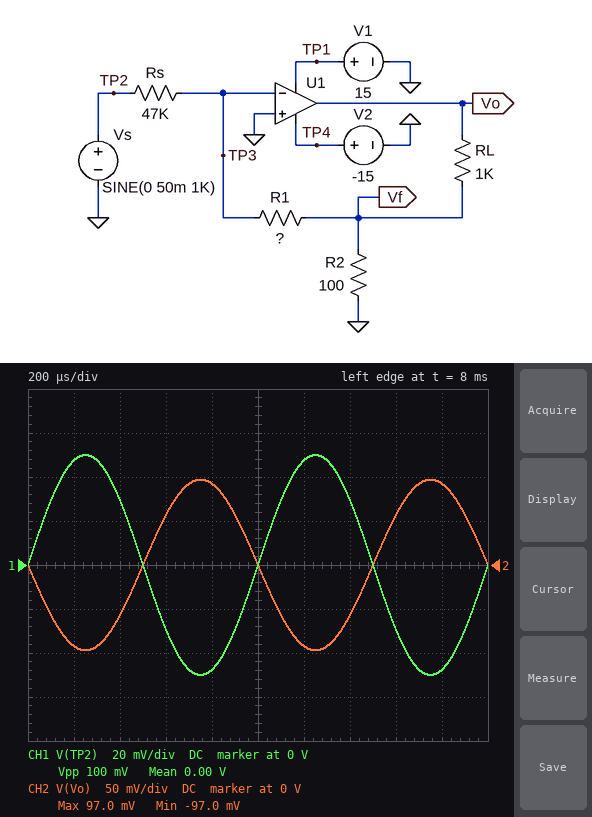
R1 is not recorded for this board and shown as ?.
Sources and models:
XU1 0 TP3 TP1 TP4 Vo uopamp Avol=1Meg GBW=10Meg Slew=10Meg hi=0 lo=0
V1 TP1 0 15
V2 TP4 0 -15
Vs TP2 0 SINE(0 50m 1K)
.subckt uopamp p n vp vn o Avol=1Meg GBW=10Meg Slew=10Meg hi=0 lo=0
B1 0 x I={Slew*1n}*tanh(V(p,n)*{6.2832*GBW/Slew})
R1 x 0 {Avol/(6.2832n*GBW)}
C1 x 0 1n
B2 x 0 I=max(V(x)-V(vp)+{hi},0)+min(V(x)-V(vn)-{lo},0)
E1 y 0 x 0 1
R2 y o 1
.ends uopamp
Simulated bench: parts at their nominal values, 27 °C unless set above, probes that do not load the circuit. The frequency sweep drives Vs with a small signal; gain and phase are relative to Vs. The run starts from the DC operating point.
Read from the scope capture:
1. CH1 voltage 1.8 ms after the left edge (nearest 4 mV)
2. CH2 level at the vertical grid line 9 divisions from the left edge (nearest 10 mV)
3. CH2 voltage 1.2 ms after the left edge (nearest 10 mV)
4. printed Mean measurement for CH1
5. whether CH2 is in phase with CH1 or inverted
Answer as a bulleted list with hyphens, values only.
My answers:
- -48 mV
- 90 mV
- -90 mV
- 0.00 V
- inverted
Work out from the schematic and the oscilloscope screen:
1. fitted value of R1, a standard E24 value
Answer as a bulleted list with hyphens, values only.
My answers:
- 8.2 kΩ
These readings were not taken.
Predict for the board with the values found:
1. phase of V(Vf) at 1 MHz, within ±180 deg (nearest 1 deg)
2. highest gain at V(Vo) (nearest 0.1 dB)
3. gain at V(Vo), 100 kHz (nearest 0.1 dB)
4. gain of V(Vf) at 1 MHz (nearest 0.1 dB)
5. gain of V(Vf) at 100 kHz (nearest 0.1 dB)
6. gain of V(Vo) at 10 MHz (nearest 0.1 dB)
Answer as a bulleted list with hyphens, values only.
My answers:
- 127 deg
- 5.8 dB
- 5.7 dB
- -19.4 dB
- -15.2 dB
- -16.5 dB
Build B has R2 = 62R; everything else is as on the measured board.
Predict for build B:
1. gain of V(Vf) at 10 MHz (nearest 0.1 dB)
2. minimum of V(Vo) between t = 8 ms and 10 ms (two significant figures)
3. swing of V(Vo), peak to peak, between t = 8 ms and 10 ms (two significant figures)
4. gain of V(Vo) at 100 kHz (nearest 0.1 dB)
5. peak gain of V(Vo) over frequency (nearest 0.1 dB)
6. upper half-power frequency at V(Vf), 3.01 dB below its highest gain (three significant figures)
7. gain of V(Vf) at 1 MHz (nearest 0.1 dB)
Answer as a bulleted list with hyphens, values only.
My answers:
- -41.2 dB
- -150 mV
- 300 mV
- 9.4 dB
- 9.6 dB
- 496 kHz
- -22.2 dB
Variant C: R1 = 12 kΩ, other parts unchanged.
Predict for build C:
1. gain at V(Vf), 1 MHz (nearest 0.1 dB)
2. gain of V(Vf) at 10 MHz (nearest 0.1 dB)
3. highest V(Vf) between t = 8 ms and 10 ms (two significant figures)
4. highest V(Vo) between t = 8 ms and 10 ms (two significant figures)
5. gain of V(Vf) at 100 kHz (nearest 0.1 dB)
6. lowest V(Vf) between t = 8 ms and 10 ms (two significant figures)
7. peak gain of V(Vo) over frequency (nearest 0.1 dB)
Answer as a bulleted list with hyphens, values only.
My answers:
- -16.5 dB
- -34.7 dB
- 13 mV
- 140 mV
- -11.9 dB
- -13 mV
- 9.0 dB
